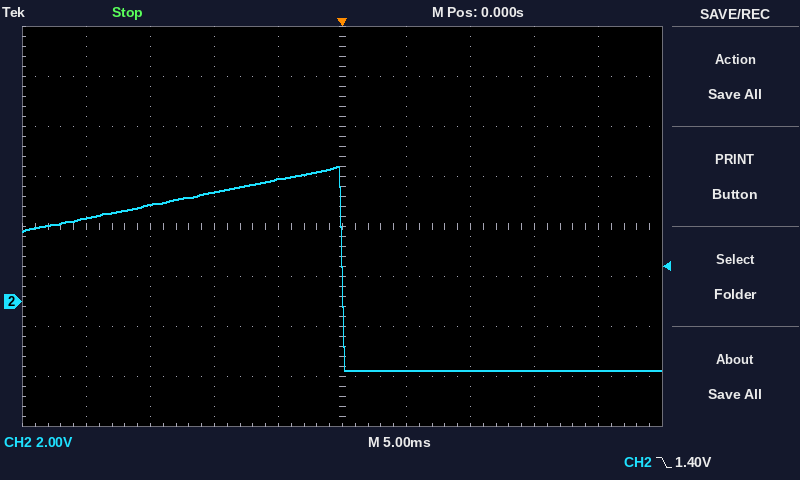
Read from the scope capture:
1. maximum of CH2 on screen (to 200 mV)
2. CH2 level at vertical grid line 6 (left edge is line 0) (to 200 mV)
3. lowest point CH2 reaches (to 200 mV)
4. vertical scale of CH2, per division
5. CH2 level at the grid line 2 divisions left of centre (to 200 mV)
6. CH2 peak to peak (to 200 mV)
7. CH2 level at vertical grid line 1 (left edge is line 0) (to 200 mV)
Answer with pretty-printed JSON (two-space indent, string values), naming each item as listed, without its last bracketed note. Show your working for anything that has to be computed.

{
  "maximum of CH2 on screen": "5.4 V",
  "CH2 level at vertical grid line 6 (left edge is line 0)": "-2.8 V",
  "lowest point CH2 reaches": "-2.8 V",
  "vertical scale of CH2, per division": "2 V",
  "CH2 level at the grid line 2 divisions left of centre": "4.4 V",
  "CH2 peak to peak": "5.4 V − (-2.8 V) = 8.2 V",
  "CH2 level at vertical grid line 1 (left edge is line 0)": "3.4 V"
}
